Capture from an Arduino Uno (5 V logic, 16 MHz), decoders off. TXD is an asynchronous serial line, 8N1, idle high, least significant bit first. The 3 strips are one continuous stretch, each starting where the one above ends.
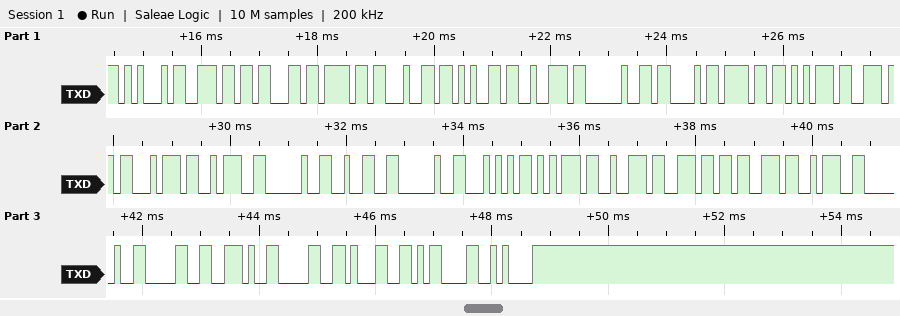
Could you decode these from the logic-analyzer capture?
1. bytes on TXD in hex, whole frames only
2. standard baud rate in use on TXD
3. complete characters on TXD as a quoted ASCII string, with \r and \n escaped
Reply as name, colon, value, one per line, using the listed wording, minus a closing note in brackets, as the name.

bytes on TXD in hex, whole frames only: 45 6E 63 6F 64 65 72 20 43 6F 75 6E 74 3A 20 32 20 54 75 72 6E 73 3A 20 30 2E 30 31 0D 0A
standard baud rate in use on TXD: 9600 baud
complete characters on TXD as a quoted ASCII string, with \r and \n escaped: "Encoder Count: 2 Turns: 0.01\r\n"
